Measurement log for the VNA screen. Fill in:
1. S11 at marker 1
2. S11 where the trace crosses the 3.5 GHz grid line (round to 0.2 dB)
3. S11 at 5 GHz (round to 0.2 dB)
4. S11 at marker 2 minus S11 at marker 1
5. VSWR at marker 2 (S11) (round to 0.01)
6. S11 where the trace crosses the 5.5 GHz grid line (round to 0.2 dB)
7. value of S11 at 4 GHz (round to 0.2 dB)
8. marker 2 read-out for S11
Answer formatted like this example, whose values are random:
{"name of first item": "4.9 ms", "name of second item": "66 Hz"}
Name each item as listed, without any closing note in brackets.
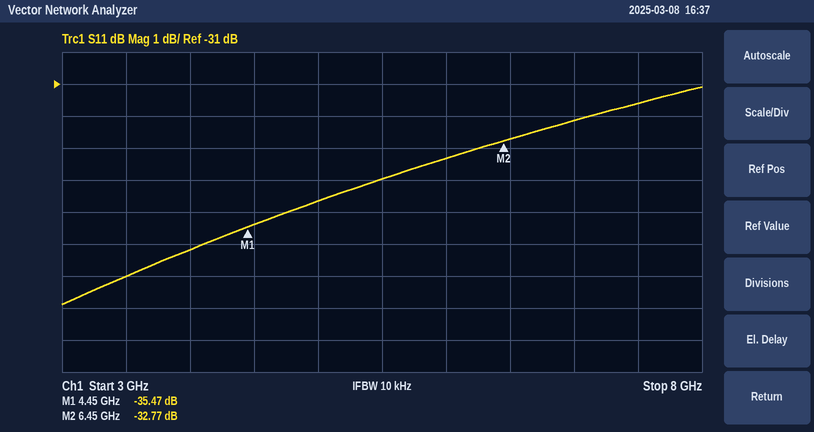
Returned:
{"S11 at marker 1": "-35.47 dB", "S11 where the trace crosses the 3.5 GHz grid line": "-37.0 dB", "S11 at 5 GHz": "-34.6 dB", "S11 at marker 2 minus S11 at marker 1": "2.70 dB", "VSWR at marker 2 (S11)": "1.05", "S11 where the trace crosses the 5.5 GHz grid line": "-34.0 dB", "value of S11 at 4 GHz": "-36.2 dB", "marker 2 read-out for S11": "-32.77 dB"}
